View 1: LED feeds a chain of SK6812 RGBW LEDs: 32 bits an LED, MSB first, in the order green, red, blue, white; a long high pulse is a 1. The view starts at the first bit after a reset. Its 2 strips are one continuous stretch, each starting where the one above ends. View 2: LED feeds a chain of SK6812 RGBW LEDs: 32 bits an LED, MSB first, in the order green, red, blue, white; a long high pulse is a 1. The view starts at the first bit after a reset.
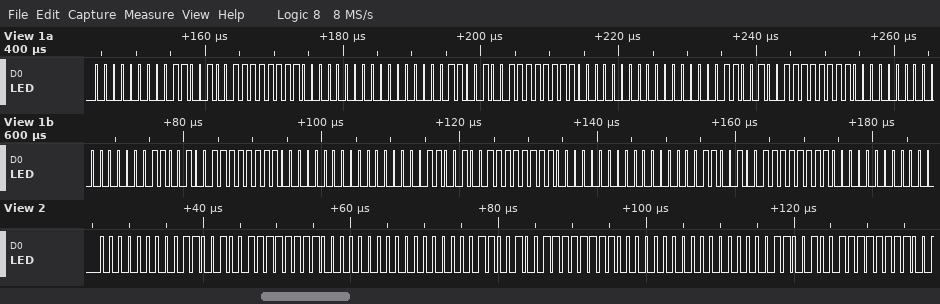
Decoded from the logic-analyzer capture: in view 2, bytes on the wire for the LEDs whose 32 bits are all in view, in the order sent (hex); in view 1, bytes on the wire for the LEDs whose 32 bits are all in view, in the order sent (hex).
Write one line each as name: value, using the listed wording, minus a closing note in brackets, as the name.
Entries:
in view 2, bytes on the wire for the LEDs whose 32 bits are all in view, in the order sent: 00 64 FF 00 00 64 FF 00
in view 1, bytes on the wire for the LEDs whose 32 bits are all in view, in the order sent: 00 64 FF 00 00 64 FF 00 00 64 FF 00 00 64 FF 00 00 64 FF 00 00 64 FF 00
